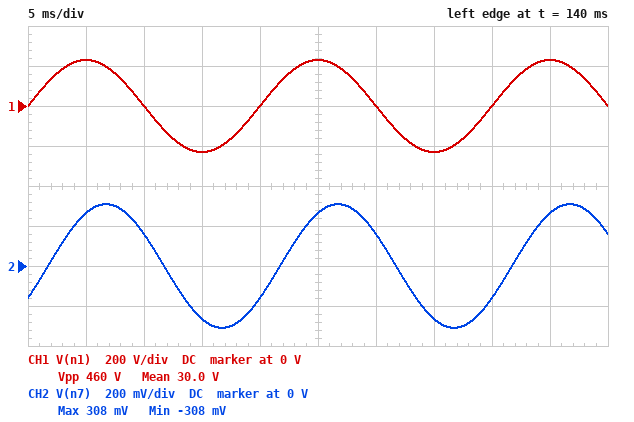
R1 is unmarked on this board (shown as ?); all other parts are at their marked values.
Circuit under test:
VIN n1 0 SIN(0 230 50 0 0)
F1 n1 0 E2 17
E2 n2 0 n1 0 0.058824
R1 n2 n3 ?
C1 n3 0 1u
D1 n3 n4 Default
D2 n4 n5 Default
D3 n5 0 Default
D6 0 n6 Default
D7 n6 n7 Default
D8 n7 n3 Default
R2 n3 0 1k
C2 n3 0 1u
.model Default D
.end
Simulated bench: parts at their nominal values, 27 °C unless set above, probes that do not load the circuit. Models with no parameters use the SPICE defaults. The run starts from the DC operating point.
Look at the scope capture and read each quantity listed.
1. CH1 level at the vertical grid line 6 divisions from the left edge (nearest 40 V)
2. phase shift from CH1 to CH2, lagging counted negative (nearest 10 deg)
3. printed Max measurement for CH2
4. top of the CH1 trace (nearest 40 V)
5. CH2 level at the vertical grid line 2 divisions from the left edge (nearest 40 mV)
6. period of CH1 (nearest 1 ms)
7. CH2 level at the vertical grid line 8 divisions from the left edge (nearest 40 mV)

0 V
-30 deg
308 mV
240 V
160 mV
20 ms
-160 mV
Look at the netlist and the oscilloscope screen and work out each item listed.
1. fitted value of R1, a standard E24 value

24 kΩ
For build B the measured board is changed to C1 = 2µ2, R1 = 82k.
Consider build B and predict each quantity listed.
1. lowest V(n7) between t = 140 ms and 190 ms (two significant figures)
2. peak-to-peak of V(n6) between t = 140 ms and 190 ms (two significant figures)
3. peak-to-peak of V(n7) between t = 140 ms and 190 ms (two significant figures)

-77 mV
77 mV
150 mV
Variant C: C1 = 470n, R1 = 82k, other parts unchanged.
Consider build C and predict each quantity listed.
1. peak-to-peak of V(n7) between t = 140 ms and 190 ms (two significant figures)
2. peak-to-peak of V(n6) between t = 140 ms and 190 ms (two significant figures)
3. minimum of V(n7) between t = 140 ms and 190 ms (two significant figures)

200 mV
99 mV
-99 mV
